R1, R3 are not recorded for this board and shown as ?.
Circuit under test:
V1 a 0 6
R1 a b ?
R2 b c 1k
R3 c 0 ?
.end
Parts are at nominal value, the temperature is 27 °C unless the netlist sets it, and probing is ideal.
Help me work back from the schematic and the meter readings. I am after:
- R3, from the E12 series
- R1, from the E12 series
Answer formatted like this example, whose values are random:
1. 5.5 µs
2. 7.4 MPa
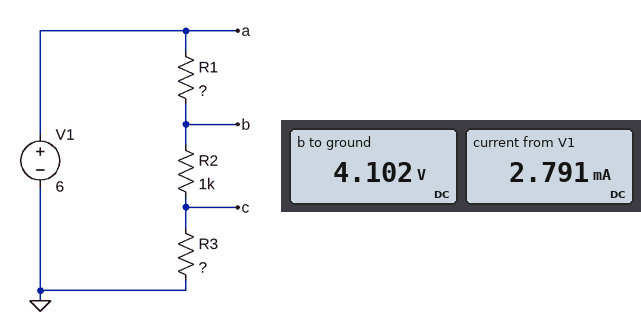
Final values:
1. 470 Ω
2. 680 Ω
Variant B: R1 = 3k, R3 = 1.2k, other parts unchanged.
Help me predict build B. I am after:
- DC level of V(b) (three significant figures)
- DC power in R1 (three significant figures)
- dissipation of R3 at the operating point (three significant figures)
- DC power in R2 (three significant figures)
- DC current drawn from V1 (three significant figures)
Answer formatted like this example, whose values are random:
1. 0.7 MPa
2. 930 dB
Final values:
1. 2.54 V
2. 3.99 mW
3. 1.60 mW
4. 1.33 mW
5. 1.15 mA
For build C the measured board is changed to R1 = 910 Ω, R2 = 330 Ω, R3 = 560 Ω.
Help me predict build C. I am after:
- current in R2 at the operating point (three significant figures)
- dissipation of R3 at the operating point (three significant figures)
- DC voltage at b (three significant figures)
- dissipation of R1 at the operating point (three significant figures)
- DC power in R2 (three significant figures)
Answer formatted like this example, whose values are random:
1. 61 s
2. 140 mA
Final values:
1. 3.33 mA
2. 6.22 mW
3. 2.97 V
4. 10.1 mW
5. 3.67 mW
